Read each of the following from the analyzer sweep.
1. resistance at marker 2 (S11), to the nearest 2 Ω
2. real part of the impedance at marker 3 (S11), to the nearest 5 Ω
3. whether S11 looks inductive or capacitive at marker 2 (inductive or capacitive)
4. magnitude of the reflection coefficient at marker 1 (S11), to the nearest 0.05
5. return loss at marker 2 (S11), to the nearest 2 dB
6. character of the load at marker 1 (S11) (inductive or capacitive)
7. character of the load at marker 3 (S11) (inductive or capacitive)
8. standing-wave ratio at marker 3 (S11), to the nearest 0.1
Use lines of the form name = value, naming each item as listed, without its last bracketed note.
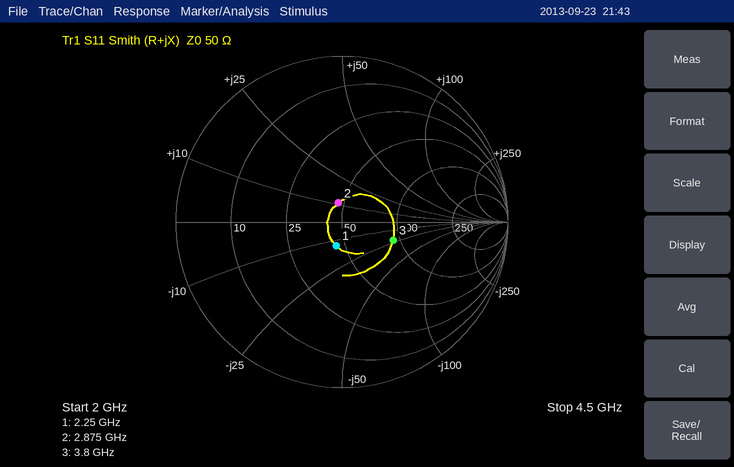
resistance at marker 2 (S11), to the nearest 2 Ω = 46 Ω
real part of the impedance at marker 3 (S11), to the nearest 5 Ω = 90 Ω
whether S11 looks inductive or capacitive at marker 2 = inductive
magnitude of the reflection coefficient at marker 1 (S11), to the nearest 0.05 = 0.15
return loss at marker 2 (S11), to the nearest 2 dB = 18 dB
character of the load at marker 1 (S11) = capacitive
character of the load at marker 3 (S11) = capacitive
standing-wave ratio at marker 3 (S11), to the nearest 0.1 = 2.0
